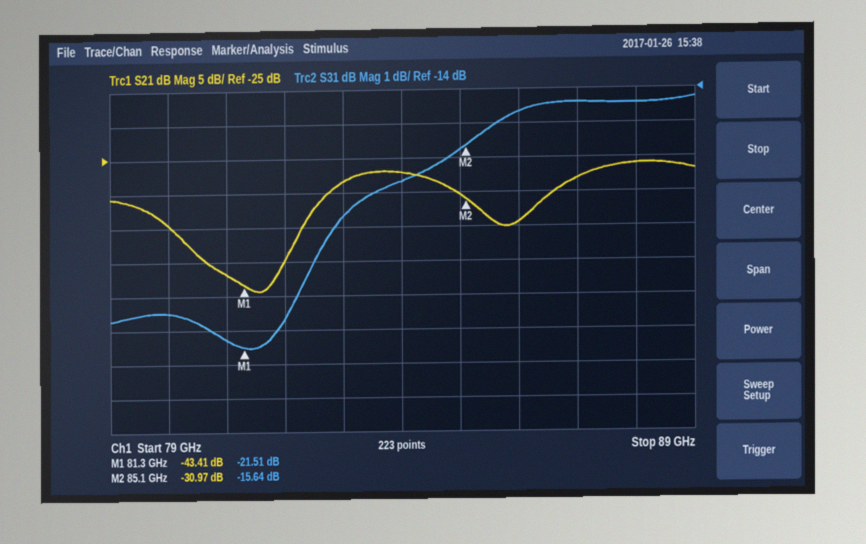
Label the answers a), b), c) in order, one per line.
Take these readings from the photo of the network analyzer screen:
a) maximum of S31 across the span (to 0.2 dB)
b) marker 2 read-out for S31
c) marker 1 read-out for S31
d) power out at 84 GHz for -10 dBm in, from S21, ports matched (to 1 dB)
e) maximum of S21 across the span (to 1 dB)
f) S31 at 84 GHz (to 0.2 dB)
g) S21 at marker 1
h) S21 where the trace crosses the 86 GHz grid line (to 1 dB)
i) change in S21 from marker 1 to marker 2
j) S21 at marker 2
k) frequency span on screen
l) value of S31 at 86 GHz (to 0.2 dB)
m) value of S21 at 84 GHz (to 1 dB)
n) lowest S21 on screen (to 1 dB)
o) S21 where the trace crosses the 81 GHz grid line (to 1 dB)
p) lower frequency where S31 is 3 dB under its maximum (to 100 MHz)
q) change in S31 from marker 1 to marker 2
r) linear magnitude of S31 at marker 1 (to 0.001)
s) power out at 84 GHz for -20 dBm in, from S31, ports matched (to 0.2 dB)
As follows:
a) -14.2 dB
b) -15.64 dB
c) -21.51 dB
d) -37 dBm
e) -26 dB
f) -16.6 dB
g) -43.41 dB
h) -34 dB
i) 12.44 dB
j) -30.97 dB
k) 10 GHz
l) -14.6 dB
m) -27 dB
n) -44 dB
o) -42 dB
p) 83.3 GHz
q) 5.87 dB
r) 0.084
s) -36.6 dBm
